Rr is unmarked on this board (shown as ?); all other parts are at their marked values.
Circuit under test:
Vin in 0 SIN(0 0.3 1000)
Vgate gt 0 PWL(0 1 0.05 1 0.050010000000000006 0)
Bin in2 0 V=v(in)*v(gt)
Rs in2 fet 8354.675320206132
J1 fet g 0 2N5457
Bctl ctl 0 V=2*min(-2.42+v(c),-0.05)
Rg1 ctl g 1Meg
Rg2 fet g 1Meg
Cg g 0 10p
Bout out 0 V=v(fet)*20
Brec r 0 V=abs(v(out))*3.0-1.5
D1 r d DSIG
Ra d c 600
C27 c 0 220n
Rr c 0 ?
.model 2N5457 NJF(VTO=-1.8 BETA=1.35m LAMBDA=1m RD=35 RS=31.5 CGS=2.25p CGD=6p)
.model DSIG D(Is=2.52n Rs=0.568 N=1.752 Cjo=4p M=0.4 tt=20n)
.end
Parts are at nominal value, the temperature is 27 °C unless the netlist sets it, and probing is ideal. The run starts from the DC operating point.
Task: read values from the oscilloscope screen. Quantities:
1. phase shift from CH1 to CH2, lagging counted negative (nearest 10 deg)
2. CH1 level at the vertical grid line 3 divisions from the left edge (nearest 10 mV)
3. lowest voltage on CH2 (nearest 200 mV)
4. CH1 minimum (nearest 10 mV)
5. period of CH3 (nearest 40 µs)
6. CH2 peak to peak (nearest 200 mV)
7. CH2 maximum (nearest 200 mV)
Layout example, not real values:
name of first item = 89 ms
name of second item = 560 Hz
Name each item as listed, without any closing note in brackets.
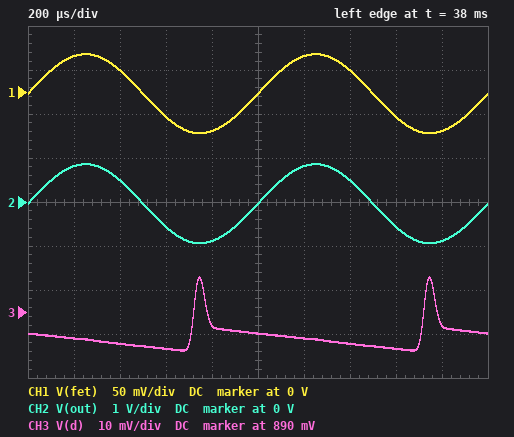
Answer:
phase shift from CH1 to CH2, lagging counted negative = 0 deg
CH1 level at the vertical grid line 3 divisions from the left edge = -30 mV
lowest voltage on CH2 = -1.0 V
CH1 minimum = -50 mV
period of CH3 = 1.00 ms
CH2 peak to peak = 1.8 V
CH2 maximum = 800 mV
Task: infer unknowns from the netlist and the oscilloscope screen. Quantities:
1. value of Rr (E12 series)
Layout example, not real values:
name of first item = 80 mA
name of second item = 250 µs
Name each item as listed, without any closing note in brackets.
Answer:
value of Rr = 680 kΩ
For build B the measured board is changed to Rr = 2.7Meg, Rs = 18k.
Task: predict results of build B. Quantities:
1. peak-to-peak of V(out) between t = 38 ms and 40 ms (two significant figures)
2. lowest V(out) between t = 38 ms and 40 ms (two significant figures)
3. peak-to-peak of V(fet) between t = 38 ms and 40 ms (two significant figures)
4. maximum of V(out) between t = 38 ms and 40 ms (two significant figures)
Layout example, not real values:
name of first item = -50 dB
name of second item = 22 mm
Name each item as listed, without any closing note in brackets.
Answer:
peak-to-peak of V(out) between t = 38 ms and 40 ms = 1.6 V
lowest V(out) between t = 38 ms and 40 ms = -870 mV
peak-to-peak of V(fet) between t = 38 ms and 40 ms = 79 mV
maximum of V(out) between t = 38 ms and 40 ms = 710 mV
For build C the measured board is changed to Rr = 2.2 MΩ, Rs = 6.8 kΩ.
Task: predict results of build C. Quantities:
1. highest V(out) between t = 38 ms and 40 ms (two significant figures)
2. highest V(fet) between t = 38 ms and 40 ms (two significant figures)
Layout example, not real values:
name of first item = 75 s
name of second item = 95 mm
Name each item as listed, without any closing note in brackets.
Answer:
highest V(out) between t = 38 ms and 40 ms = 880 mV
highest V(fet) between t = 38 ms and 40 ms = 44 mV
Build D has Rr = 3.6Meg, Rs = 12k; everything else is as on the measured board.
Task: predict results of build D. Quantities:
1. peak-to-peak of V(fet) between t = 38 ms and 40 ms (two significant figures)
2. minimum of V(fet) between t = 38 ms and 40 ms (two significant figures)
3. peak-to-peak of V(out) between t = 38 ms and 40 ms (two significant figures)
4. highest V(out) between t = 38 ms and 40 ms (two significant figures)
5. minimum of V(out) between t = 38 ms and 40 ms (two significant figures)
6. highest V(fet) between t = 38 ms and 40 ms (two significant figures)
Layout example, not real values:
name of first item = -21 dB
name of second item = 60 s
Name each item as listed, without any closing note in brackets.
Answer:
peak-to-peak of V(fet) between t = 38 ms and 40 ms = 83 mV
minimum of V(fet) between t = 38 ms and 40 ms = -44 mV
peak-to-peak of V(out) between t = 38 ms and 40 ms = 1.7 V
highest V(out) between t = 38 ms and 40 ms = 780 mV
minimum of V(out) between t = 38 ms and 40 ms = -890 mV
highest V(fet) between t = 38 ms and 40 ms = 39 mV
